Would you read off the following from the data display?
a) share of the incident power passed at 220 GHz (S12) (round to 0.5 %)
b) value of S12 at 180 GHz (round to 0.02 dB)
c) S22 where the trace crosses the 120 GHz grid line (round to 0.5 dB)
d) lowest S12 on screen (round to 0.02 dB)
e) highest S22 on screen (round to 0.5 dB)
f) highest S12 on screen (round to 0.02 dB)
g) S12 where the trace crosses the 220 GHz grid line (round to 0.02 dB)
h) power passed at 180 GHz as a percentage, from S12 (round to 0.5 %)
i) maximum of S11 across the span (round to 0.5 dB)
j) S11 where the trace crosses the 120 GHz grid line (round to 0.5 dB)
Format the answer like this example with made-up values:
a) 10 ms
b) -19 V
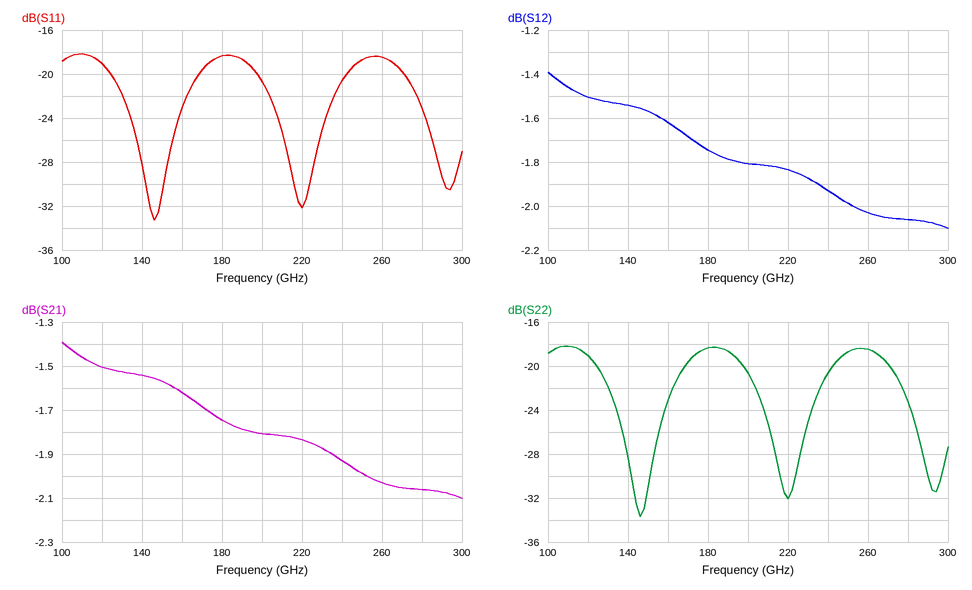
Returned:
a) 65.5 %
b) -1.74 dB
c) -19.0 dB
d) -2.10 dB
e) -18.0 dB
f) -1.40 dB
g) -1.84 dB
h) 67.0 %
i) -18.0 dB
j) -19.0 dB
